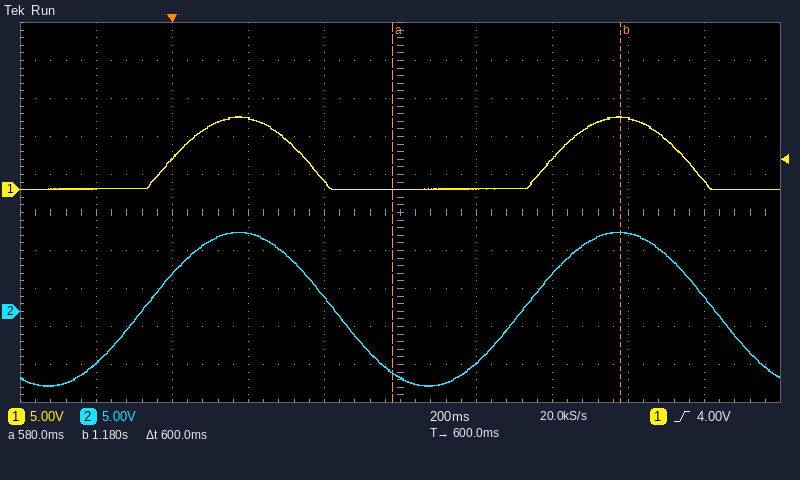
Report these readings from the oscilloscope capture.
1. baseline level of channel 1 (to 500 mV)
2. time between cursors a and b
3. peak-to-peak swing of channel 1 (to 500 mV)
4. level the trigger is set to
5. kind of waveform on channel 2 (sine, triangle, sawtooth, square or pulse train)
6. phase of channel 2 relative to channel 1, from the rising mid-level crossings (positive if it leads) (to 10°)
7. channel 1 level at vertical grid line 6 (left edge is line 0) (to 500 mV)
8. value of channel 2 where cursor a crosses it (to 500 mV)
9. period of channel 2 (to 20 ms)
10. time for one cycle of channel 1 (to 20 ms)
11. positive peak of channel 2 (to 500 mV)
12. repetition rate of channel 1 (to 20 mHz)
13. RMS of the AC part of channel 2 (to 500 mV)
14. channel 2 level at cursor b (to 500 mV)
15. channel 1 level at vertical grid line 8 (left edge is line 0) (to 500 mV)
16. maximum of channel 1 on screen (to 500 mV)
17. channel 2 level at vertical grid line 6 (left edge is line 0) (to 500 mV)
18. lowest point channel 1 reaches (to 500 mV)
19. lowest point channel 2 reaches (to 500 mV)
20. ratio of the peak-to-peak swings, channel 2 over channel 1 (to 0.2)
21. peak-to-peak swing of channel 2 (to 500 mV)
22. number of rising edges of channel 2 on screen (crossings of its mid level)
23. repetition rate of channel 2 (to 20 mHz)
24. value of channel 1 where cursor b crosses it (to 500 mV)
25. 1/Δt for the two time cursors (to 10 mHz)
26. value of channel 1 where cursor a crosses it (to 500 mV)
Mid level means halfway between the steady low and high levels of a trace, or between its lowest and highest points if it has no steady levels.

0.0 V
600 ms
9.5 V
4.00 V
sine
+30°
0.0 V
-8.0 V
1.00 s
1.00 s
10.5 V
1.00 Hz
7.0 V
10.5 V
9.5 V
9.5 V
-7.0 V
0.0 V
-10.0 V
2.2
20.5 V
2
1.00 Hz
9.5 V
1.67 Hz
0.0 V
